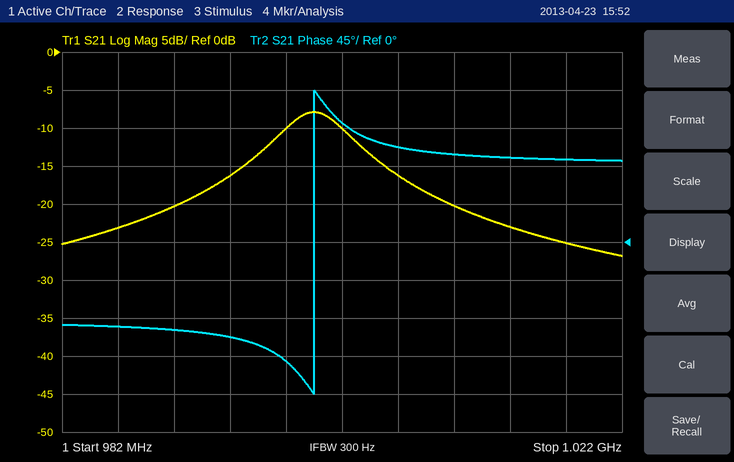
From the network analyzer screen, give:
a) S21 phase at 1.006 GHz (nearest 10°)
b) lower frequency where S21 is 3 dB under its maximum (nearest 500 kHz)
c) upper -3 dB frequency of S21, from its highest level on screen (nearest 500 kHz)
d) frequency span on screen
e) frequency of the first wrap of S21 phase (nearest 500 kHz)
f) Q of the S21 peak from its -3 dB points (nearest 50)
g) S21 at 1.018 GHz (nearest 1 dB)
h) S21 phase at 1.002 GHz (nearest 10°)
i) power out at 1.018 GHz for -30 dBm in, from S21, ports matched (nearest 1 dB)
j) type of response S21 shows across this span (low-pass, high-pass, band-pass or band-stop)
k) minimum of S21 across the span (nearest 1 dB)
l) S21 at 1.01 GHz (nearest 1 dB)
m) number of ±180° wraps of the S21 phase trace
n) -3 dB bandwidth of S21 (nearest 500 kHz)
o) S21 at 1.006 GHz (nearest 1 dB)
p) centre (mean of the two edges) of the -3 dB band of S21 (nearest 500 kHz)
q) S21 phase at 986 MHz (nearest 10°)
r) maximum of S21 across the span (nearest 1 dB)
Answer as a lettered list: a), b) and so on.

a) 110°
b) 997.5 MHz
c) 1.0025 GHz
d) 40 MHz
e) 1.0000 GHz
f) 200
g) -25 dB
h) 140°
i) -55 dBm
j) band-pass
k) -27 dB
l) -20 dB
m) 1
n) 5.0 MHz
o) -16 dB
p) 1.0000 GHz
q) -100°
r) -8 dB
